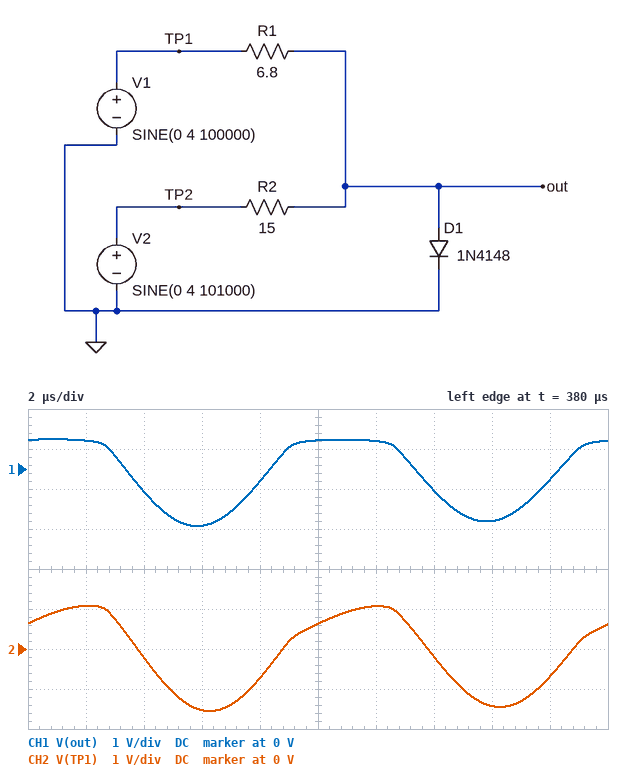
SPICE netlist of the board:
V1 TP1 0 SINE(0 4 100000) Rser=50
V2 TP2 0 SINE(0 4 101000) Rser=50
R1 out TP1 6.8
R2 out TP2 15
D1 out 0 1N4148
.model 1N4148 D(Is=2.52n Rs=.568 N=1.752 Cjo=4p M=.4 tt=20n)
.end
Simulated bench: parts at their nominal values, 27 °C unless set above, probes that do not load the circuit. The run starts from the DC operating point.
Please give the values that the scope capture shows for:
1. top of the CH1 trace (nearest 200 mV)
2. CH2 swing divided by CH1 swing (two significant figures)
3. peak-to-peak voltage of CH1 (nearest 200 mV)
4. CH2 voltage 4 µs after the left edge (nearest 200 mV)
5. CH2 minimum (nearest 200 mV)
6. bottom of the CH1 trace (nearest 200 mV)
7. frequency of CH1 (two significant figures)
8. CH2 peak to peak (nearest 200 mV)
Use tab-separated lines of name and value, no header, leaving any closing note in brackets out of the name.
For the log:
top of the CH1 trace	800 mV
CH2 swing divided by CH1 swing	1.2
peak-to-peak voltage of CH1	2.2 V
CH2 voltage 4 µs after the left edge	-200 mV
CH2 minimum	-1.6 V
bottom of the CH1 trace	-1.4 V
frequency of CH1	100 kHz
CH2 peak to peak	2.6 V
